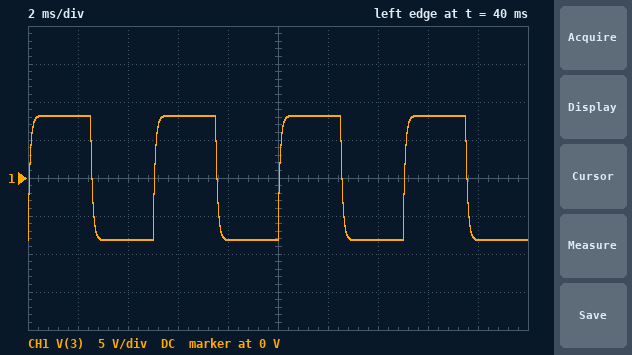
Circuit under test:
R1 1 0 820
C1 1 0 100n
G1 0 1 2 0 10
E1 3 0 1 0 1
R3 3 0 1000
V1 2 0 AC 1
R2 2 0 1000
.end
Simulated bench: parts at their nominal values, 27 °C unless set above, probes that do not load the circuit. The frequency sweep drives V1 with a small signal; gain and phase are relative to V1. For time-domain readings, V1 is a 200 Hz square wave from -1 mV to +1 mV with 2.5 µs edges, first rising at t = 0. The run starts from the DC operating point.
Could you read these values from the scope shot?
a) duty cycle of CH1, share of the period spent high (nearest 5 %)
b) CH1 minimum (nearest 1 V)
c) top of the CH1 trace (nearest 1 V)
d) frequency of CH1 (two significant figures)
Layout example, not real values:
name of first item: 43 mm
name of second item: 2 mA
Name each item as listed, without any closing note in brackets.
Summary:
duty cycle of CH1, share of the period spent high: 50 %
CH1 minimum: -8 V
top of the CH1 trace: 8 V
frequency of CH1: 200 Hz
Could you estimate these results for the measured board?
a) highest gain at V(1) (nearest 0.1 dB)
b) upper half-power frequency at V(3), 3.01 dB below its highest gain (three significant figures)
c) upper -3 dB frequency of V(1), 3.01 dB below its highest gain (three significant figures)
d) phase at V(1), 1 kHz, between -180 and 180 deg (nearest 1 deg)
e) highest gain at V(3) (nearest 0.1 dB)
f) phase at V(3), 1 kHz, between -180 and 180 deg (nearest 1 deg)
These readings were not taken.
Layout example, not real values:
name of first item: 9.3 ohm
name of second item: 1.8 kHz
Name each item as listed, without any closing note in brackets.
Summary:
highest gain at V(1): 78.3 dB
upper half-power frequency at V(3), 3.01 dB below its highest gain: 1.94 kHz
upper -3 dB frequency of V(1), 3.01 dB below its highest gain: 1.94 kHz
phase at V(1), 1 kHz, between -180 and 180 deg: -27 deg
highest gain at V(3): 78.3 dB
phase at V(3), 1 kHz, between -180 and 180 deg: -27 deg
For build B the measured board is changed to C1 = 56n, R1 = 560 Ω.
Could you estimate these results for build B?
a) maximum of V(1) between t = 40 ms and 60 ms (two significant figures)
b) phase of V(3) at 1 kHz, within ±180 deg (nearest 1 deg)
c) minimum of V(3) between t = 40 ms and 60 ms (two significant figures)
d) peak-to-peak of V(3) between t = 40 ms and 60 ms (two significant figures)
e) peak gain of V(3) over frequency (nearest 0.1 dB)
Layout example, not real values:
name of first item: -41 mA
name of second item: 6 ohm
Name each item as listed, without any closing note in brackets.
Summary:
maximum of V(1) between t = 40 ms and 60 ms: 5.6 V
phase of V(3) at 1 kHz, within ±180 deg: -11 deg
minimum of V(3) between t = 40 ms and 60 ms: -5.6 V
peak-to-peak of V(3) between t = 40 ms and 60 ms: 11 V
peak gain of V(3) over frequency: 75.0 dB
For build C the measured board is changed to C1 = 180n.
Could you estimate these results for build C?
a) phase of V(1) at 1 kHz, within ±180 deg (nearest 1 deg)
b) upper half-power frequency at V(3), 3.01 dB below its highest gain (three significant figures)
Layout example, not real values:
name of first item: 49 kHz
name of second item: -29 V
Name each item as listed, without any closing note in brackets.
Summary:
phase of V(1) at 1 kHz, within ±180 deg: -43 deg
upper half-power frequency at V(3), 3.01 dB below its highest gain: 1.08 kHz
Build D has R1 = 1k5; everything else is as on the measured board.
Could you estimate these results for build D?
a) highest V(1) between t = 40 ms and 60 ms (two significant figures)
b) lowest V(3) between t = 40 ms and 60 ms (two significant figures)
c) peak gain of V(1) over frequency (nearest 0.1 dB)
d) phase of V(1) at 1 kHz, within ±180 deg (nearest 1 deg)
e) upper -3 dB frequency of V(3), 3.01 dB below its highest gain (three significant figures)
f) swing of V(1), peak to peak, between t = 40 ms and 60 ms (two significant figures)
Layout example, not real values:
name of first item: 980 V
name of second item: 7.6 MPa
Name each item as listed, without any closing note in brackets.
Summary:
highest V(1) between t = 40 ms and 60 ms: 15 V
lowest V(3) between t = 40 ms and 60 ms: -15 V
peak gain of V(1) over frequency: 83.5 dB
phase of V(1) at 1 kHz, within ±180 deg: -43 deg
upper -3 dB frequency of V(3), 3.01 dB below its highest gain: 1.06 kHz
swing of V(1), peak to peak, between t = 40 ms and 60 ms: 30 V
